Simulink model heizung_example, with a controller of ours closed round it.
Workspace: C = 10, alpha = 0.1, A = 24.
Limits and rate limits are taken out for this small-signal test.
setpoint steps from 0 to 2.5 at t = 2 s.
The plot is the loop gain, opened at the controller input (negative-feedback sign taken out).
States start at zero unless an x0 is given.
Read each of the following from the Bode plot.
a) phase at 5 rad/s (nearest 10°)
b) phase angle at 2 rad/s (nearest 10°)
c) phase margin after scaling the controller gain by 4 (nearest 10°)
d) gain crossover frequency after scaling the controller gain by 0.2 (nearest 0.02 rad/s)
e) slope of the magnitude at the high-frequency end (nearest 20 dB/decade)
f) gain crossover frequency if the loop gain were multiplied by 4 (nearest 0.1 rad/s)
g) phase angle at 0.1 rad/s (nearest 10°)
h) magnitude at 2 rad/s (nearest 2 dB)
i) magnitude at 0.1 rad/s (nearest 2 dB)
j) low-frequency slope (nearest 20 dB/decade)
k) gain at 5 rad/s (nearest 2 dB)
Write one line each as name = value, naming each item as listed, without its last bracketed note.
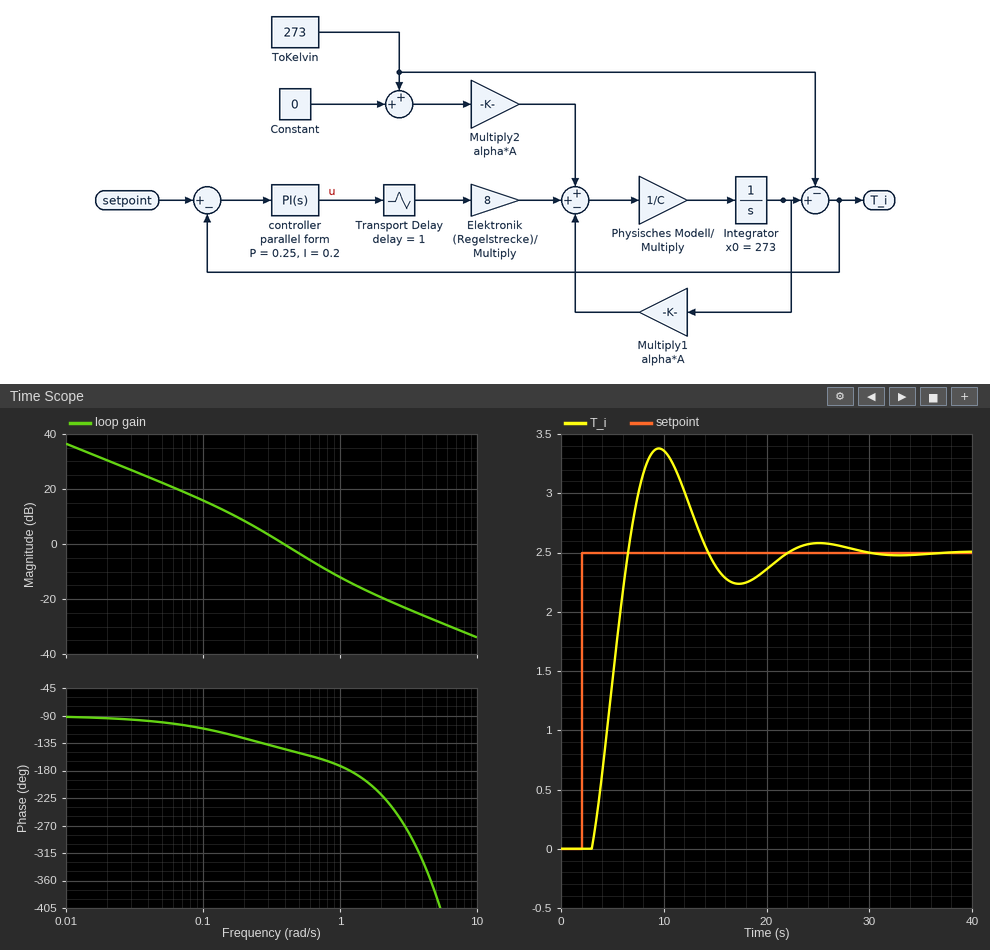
phase at 5 rad/s = -380°
phase angle at 2 rad/s = -220°
phase margin after scaling the controller gain by 4 = 10°
gain crossover frequency after scaling the controller gain by 0.2 = 0.12 rad/s
slope of the magnitude at the high-frequency end = -20 dB/decade
gain crossover frequency if the loop gain were multiplied by 4 = 1.0 rad/s
phase angle at 0.1 rad/s = -110°
magnitude at 2 rad/s = -20 dB
magnitude at 0.1 rad/s = 16 dB
low-frequency slope = -20 dB/decade
gain at 5 rad/s = -28 dB
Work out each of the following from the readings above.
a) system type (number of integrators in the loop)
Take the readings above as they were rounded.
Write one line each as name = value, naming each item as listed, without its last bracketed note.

system type = 1
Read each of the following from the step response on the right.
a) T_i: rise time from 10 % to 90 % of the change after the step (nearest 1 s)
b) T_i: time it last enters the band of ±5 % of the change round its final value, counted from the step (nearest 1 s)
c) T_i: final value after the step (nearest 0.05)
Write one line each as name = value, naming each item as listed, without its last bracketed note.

T_i: rise time from 10 % to 90 % of the change after the step = 3 s
T_i: time it last enters the band of ±5 % of the change round its final value, counted from the step = 18 s
T_i: final value after the step = 2.50
